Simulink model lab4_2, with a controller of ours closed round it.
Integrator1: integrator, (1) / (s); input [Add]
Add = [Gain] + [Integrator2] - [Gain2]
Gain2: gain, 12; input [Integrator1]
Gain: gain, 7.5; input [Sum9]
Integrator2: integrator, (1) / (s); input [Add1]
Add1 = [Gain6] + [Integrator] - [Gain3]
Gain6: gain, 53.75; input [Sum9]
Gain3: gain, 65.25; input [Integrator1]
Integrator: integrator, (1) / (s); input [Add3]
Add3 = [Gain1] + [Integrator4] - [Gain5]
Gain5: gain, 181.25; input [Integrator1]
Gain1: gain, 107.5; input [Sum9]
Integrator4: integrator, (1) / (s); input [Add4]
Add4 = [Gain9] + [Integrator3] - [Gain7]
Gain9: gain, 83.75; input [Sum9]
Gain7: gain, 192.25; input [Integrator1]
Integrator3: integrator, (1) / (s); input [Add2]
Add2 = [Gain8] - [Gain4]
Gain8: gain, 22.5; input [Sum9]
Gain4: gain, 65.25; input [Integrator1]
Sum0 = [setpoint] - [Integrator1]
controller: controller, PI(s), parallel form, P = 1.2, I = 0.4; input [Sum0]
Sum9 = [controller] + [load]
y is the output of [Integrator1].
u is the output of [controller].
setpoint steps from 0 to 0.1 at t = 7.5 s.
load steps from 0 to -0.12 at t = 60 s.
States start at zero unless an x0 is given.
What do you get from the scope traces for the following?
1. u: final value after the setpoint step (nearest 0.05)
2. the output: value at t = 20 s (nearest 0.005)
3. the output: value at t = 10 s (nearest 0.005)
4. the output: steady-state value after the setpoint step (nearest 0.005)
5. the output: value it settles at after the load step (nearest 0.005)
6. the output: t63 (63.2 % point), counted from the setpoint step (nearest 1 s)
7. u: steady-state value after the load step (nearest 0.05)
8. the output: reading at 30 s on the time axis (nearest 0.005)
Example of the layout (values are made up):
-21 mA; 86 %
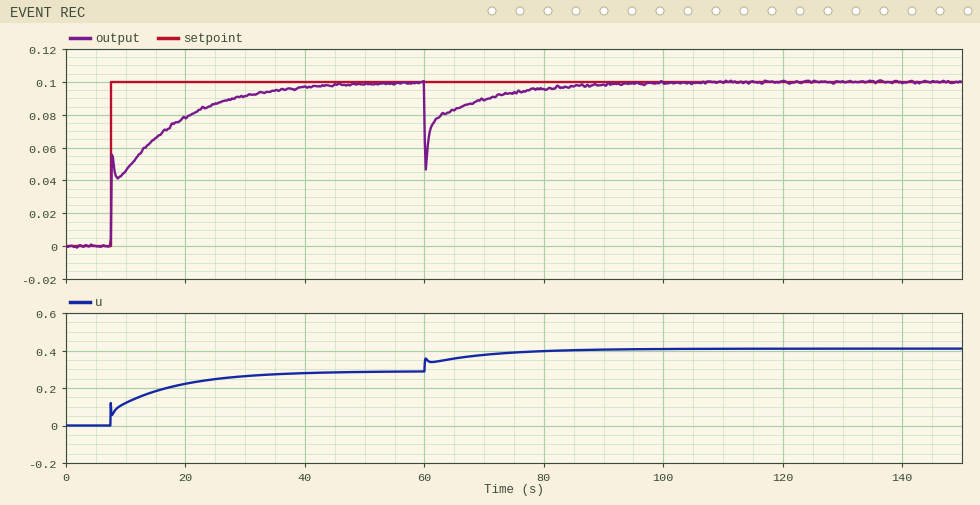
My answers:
0.30; 0.080; 0.045; 0.100; 0.100; 7 s; 0.40; 0.090
